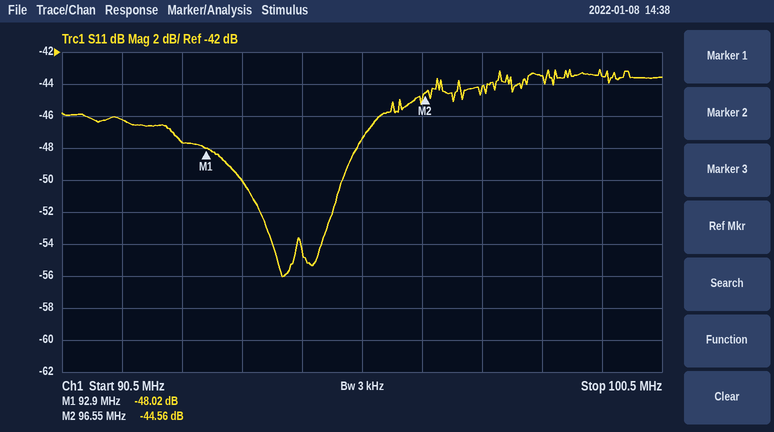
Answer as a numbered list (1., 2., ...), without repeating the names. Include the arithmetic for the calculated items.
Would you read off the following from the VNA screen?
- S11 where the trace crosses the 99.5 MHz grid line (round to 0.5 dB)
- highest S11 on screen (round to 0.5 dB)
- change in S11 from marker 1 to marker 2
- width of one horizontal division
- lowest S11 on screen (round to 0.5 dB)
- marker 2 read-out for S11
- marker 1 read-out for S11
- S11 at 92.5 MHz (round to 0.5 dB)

1. -43.5 dB
2. -43.0 dB
3. -44.56 − (-48.02) = 3.46 dB
4. 1 MHz
5. -56.0 dB
6. -44.56 dB
7. -48.02 dB
8. -47.5 dB
